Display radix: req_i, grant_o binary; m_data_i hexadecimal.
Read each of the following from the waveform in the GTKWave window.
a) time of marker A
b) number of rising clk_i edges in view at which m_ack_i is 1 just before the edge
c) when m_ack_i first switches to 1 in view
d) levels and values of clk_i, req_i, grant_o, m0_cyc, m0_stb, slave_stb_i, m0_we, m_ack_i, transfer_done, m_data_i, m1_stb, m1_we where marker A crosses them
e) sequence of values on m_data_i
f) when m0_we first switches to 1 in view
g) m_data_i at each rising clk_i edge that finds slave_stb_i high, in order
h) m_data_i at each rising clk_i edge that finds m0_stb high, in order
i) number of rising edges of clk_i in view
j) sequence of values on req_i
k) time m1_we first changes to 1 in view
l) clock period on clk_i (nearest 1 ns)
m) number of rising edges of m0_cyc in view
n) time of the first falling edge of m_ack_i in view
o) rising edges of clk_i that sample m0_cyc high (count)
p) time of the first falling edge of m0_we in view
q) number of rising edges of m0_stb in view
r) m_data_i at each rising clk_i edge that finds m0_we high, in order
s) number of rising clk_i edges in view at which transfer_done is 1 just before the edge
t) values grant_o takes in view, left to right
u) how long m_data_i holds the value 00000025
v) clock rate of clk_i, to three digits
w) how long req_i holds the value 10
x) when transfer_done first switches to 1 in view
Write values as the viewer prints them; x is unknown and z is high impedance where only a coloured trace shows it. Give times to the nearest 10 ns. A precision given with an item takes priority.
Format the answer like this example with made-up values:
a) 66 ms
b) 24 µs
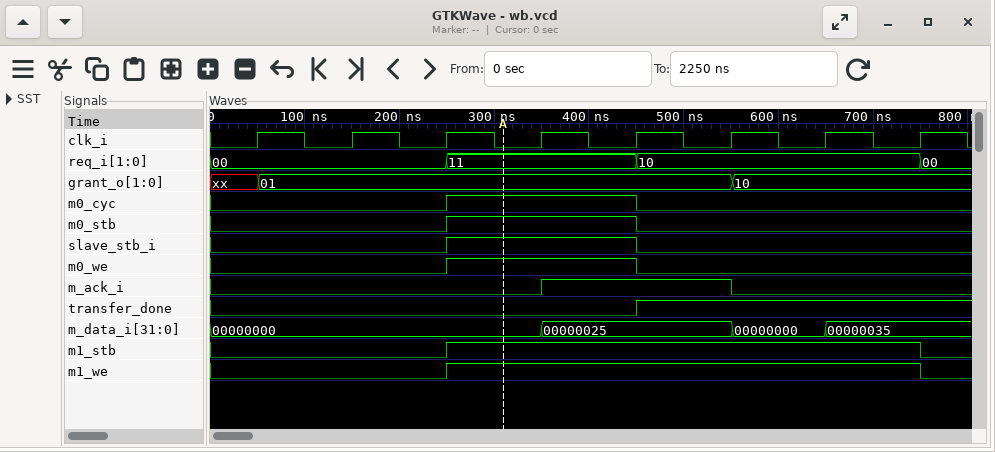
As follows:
a) 310 ns
b) 2
c) 350 ns
d) clk_i=0, req_i=11, grant_o=01, m0_cyc=1, m0_stb=1, slave_stb_i=1, m0_we=1, m_ack_i=0, transfer_done=0, m_data_i=00000000, m1_stb=1, m1_we=1
e) 00000000, 00000025, 00000000, 00000035
f) 250 ns
g) 00000000, 00000025
h) 00000000, 00000025
i) 8
j) 00, 11, 10, 00
k) 250 ns
l) 100 ns
m) 1
n) 550 ns
o) 2
p) 450 ns
q) 1
r) 00000000, 00000025
s) 3
t) xx, 01, 10
u) 200 ns
v) 10.0 MHz
w) 300 ns
x) 450 ns
